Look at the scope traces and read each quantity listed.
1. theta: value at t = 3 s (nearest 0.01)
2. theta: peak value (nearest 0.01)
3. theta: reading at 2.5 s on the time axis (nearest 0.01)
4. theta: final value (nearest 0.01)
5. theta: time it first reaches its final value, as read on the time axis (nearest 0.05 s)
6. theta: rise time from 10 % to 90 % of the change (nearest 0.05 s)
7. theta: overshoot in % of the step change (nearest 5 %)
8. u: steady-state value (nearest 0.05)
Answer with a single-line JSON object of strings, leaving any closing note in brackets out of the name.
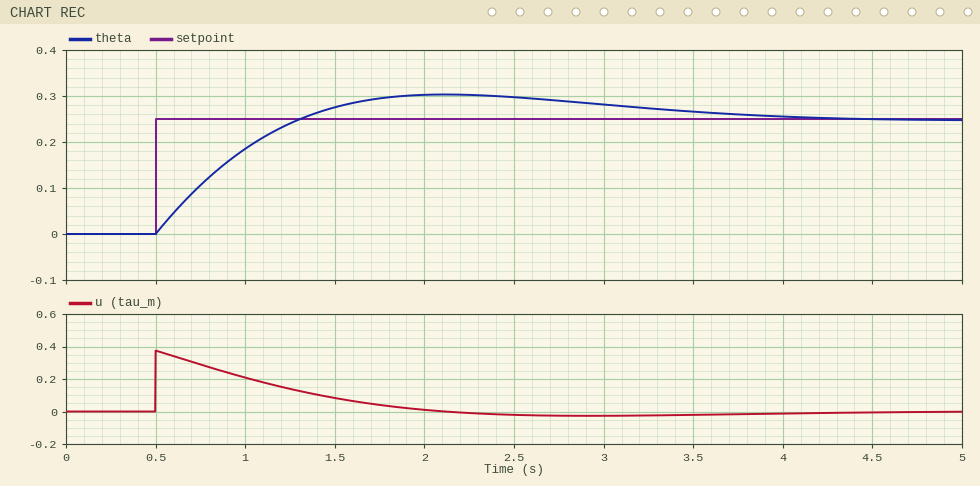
{"theta: value at t = 3 s": "0.28", "theta: peak value": "0.30", "theta: reading at 2.5 s on the time axis": "0.30", "theta: final value": "0.25", "theta: time it first reaches its final value, as read on the time axis": "1.30 s", "theta: rise time from 10 % to 90 % of the change": "0.60 s", "theta: overshoot in % of the step change": "20 %", "u: steady-state value": "0.00"}
